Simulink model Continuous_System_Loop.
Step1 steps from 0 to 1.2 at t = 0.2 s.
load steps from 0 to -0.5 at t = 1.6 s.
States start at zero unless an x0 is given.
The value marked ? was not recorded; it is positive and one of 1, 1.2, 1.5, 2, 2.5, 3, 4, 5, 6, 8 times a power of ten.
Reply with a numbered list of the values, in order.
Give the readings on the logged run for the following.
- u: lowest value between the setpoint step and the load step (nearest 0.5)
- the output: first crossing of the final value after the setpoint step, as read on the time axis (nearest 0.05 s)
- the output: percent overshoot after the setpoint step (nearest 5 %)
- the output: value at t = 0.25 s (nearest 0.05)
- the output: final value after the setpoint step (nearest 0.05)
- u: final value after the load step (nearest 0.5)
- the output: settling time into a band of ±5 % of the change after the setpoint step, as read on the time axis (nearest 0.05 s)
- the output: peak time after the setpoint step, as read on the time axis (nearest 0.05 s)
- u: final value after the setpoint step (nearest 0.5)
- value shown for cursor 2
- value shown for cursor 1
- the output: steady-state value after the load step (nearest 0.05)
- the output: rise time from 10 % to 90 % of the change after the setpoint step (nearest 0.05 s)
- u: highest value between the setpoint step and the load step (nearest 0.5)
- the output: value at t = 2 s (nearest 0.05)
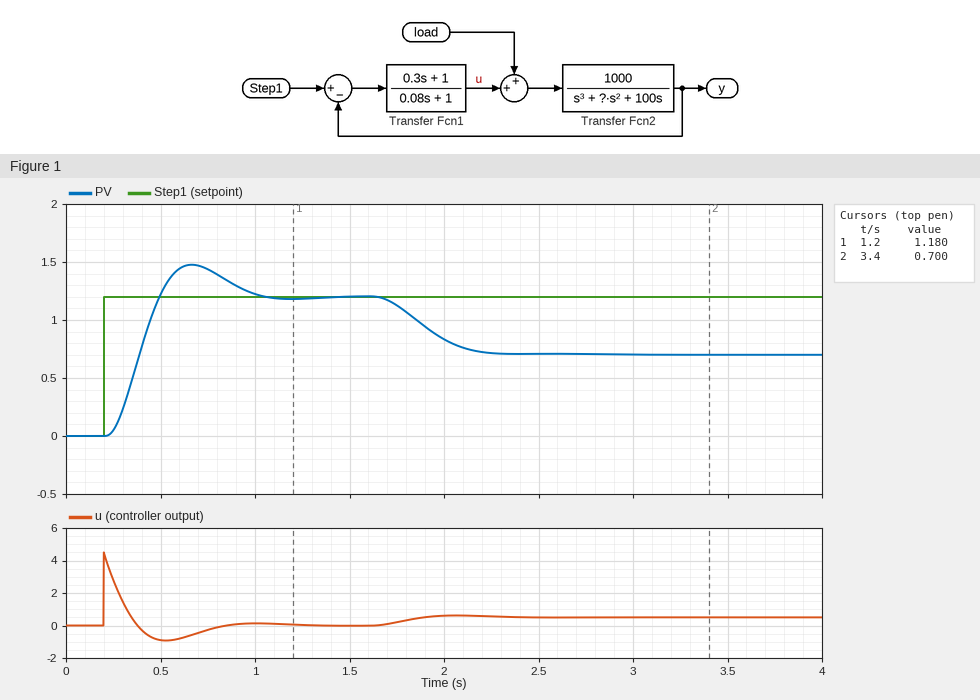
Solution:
1. -1.0
2. 0.50 s
3. 25 %
4. 0.05
5. 1.20
6. 0.5
7. 0.95 s
8. 0.65 s
9. 0.0
10. 0.700
11. 1.180
12. 0.70
13. 0.20 s
14. 4.5
15. 0.85
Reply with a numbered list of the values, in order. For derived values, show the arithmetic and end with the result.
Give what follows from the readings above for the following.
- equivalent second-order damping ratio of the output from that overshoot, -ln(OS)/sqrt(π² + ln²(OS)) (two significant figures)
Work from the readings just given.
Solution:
1. ln(0.25) = -1.386; 1.386 / sqrt(9.870 + 1.922) = 0.40
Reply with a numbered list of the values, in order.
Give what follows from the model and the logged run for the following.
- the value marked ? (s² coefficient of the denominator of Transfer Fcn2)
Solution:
1. 50
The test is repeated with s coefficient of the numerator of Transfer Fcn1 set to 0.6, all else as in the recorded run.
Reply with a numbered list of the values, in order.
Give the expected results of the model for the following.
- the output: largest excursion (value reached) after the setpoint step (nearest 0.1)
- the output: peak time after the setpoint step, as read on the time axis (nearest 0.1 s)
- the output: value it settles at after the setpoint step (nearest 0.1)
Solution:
1. 1.5
2. 0.5 s
3. 1.2
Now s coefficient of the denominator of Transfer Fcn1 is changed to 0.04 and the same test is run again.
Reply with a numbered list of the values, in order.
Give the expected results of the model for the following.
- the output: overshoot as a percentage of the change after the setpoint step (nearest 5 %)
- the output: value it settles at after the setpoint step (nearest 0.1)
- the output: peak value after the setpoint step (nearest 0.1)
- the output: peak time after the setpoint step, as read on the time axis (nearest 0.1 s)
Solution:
1. 10 %
2. 1.2
3. 1.3
4. 0.6 s
